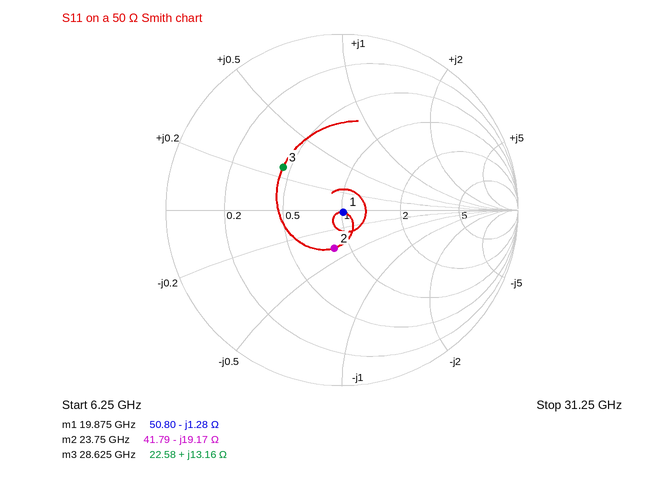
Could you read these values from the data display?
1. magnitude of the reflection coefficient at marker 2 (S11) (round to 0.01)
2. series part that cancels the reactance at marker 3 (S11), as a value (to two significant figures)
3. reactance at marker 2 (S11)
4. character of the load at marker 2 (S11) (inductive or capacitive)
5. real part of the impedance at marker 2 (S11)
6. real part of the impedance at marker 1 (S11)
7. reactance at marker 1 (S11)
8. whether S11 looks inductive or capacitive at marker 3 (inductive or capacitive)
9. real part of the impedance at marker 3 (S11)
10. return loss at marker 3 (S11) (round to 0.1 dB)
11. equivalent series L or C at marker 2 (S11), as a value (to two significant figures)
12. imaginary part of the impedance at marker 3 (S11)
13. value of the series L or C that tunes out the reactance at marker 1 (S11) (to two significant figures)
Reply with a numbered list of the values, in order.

1. 0.22
2. 420 fF
3. -19.17 Ω
4. capacitive
5. 41.79 Ω
6. 50.80 Ω
7. -1.28 Ω
8. inductive
9. 22.58 Ω
10. 7.7 dB
11. 350 fF
12. +13.16 Ω
13. 10 pH
